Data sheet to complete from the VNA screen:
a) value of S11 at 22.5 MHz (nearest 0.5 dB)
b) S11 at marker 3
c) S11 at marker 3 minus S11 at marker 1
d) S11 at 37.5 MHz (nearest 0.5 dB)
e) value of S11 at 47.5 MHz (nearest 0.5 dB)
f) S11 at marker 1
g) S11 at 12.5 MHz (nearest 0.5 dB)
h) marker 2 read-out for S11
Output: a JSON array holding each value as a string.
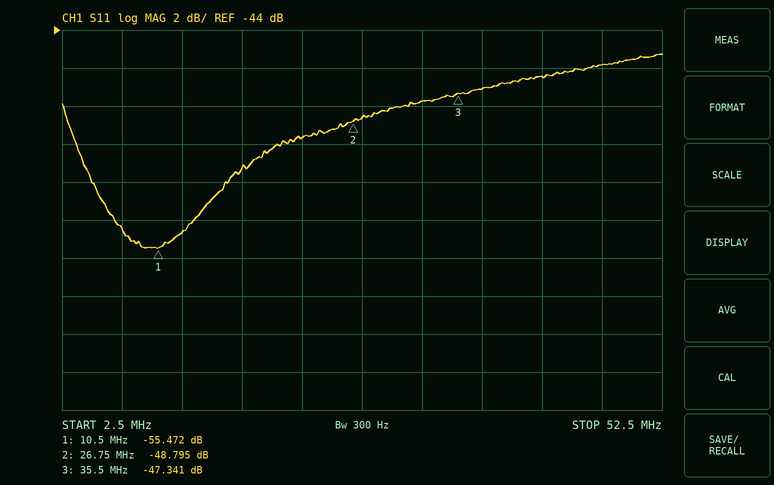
["-49.5 dB", "-47.341 dB", "8.131 dB", "-47.0 dB", "-46.0 dB", "-55.472 dB", "-54.5 dB", "-48.795 dB"]
